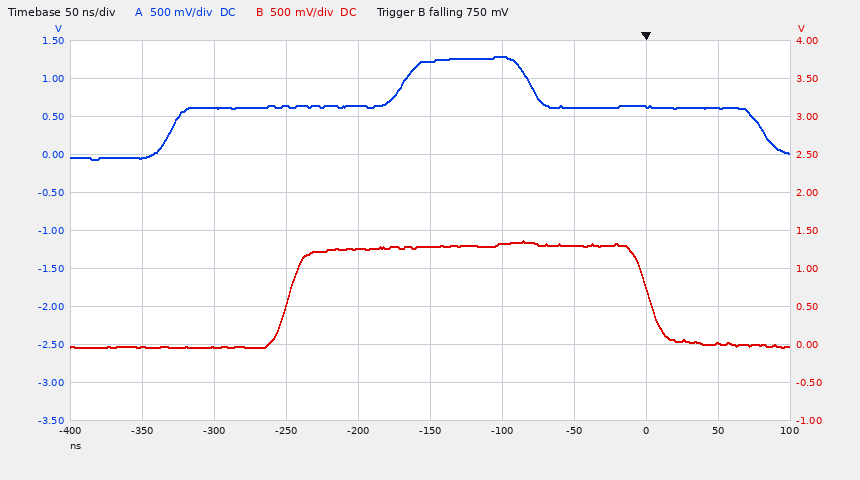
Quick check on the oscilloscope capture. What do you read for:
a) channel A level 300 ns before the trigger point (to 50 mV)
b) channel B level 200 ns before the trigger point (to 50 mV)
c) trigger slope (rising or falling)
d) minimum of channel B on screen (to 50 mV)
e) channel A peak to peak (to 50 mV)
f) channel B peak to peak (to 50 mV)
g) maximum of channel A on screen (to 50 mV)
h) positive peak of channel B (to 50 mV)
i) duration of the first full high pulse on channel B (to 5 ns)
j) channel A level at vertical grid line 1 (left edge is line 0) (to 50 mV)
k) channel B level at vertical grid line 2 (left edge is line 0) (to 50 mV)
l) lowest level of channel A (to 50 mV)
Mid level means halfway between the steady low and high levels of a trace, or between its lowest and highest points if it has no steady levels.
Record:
600 mV
1.25 V
falling
-50 mV
1.35 V
1.40 V
1.30 V
1.35 V
250 ns
-50 mV
-50 mV
-50 mV
